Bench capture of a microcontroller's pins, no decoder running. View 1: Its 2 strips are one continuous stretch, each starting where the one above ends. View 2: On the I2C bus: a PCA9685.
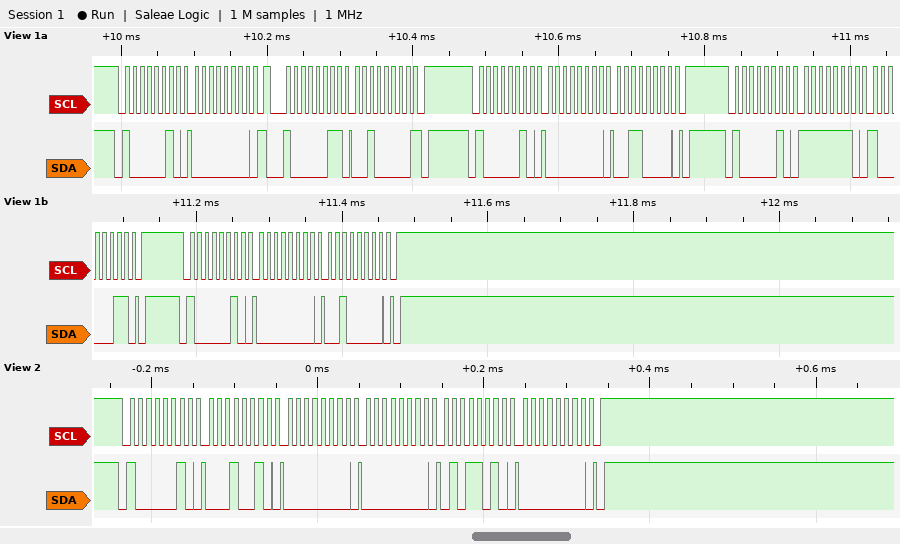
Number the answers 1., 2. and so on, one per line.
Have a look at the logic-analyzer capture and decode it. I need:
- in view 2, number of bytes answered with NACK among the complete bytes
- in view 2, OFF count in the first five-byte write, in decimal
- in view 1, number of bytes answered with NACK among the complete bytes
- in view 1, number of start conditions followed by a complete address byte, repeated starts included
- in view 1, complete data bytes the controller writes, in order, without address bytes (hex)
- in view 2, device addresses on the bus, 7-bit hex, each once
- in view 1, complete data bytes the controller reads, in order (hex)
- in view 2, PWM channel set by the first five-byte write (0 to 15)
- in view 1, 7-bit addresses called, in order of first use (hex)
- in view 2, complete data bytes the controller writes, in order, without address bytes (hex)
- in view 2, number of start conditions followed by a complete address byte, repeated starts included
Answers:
1. 0
2. 90
3. 1
4. 5
5. 00 00 30 FE 83 00 20
6. 0x41
7. 20
8. 3
9. 0x41
10. 12 00 00 5A 00
11. 1
